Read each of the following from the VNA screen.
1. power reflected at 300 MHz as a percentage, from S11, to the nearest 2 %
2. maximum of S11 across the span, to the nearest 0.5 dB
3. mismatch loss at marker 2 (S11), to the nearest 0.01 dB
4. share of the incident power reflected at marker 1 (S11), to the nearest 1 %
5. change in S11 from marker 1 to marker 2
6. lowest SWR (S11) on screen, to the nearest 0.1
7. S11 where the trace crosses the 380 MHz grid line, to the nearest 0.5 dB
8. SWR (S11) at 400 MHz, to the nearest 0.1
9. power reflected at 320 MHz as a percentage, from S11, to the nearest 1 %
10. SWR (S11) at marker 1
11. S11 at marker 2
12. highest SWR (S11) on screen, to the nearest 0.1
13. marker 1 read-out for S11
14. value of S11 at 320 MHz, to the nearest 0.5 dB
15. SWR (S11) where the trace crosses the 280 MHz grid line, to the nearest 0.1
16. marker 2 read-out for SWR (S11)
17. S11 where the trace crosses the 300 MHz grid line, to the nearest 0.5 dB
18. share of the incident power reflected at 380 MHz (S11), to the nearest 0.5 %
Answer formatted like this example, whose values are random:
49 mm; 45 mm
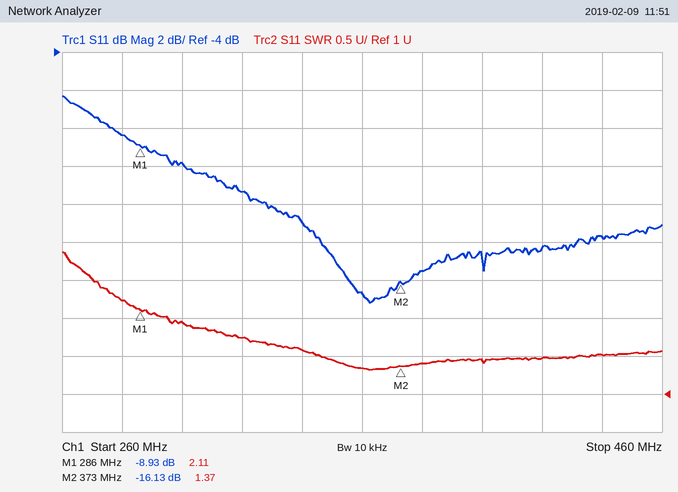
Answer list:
10 %; -6.5 dB; 0.11 dB; 13 %; -7.20 dB; 1.3; -15.5 dB; 1.4; 7 %; 2.11; -16.13 dB; 2.9; -8.93 dB; -11.5 dB; 2.2; 1.37; -10.0 dB; 3.0 %
